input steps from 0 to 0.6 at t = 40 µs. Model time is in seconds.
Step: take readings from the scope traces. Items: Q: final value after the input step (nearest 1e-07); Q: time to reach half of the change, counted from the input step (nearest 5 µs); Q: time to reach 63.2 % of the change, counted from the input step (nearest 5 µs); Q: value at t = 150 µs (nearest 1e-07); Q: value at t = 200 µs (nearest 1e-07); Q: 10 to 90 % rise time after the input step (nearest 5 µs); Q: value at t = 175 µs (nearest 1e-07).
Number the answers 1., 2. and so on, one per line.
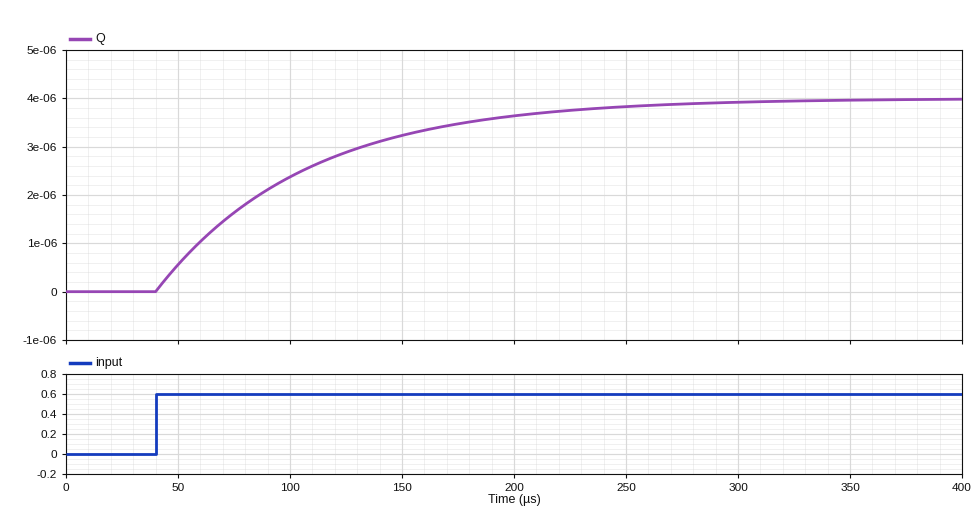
1. 0.0000040
2. 45 µs
3. 65 µs
4. 0.0000032
5. 0.0000036
6. 145 µs
7. 0.0000035
